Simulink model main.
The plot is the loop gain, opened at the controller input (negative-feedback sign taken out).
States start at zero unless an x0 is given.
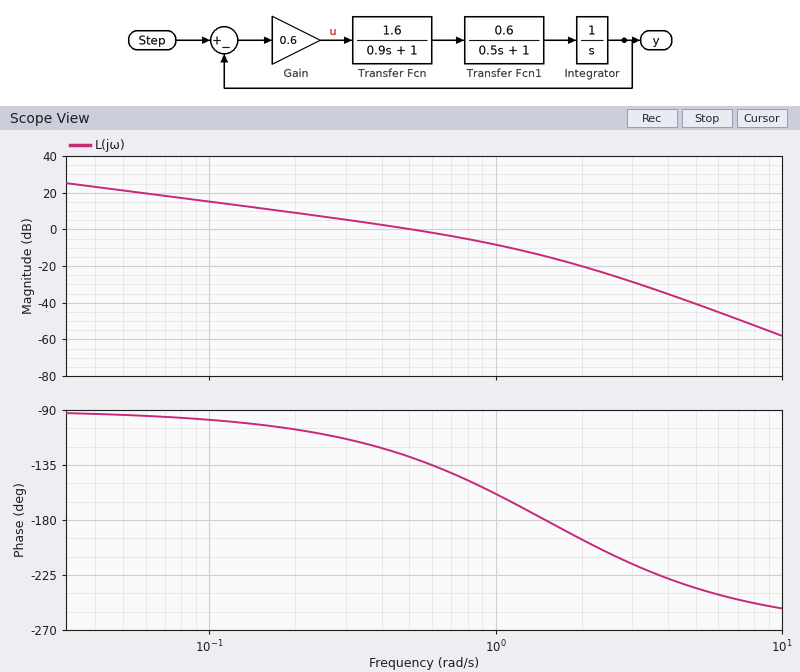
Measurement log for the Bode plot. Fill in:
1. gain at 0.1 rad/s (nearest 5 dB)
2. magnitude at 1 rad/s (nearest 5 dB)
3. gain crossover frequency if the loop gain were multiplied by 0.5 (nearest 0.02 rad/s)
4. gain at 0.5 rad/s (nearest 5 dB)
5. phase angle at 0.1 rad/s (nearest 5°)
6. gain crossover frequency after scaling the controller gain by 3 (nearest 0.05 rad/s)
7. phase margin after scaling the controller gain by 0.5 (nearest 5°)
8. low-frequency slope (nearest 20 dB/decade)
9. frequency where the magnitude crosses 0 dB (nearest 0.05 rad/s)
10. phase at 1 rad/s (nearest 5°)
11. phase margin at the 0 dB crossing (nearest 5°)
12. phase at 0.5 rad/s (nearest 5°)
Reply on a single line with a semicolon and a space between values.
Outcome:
15 dB; -10 dB; 0.28 rad/s; 0 dB; -100°; 1.10 rad/s; 70°; -20 dB/decade; 0.50 rad/s; -160°; 50°; -130°
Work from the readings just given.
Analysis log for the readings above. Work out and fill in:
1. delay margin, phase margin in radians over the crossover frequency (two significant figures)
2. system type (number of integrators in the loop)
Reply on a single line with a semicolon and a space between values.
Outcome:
1.7 s; 1
